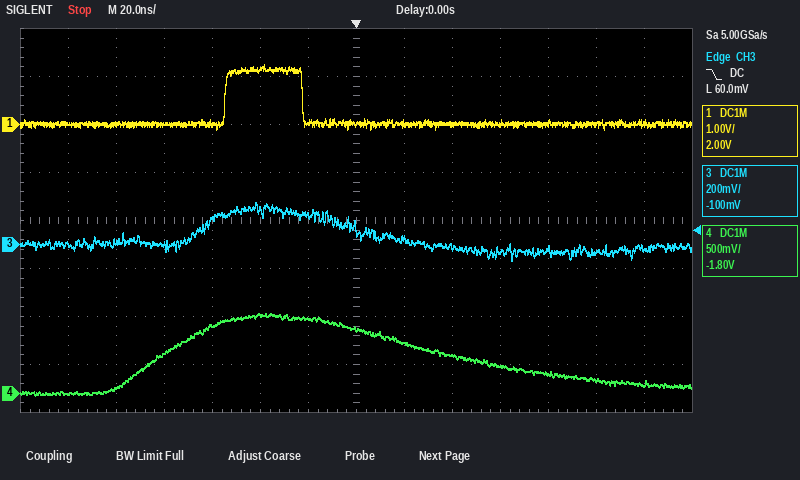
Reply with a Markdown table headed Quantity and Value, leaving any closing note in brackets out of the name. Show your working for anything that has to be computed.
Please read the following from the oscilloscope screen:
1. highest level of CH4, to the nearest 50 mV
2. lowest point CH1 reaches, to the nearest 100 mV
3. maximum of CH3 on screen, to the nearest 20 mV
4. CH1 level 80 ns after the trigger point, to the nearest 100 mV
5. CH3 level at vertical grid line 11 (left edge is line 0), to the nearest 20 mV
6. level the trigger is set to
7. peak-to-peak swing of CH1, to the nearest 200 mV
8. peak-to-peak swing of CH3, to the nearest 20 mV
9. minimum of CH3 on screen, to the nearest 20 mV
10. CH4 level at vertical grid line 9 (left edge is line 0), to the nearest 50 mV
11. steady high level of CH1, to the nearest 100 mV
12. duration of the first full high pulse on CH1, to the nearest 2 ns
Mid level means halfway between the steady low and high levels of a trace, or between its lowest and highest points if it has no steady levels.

| Quantity | Value |
|---|---|
| highest level of CH4, to the nearest 50 mV | 850 mV |
| lowest point CH1 reaches, to the nearest 100 mV | -100 mV |
| maximum of CH3 on screen, to the nearest 20 mV | 180 mV |
| CH1 level 80 ns after the trigger point, to the nearest 100 mV | 0.0 V |
| CH3 level at vertical grid line 11 (left edge is line 0), to the nearest 20 mV | -20 mV |
| level the trigger is set to | 60.0 mV |
| peak-to-peak swing of CH1, to the nearest 200 mV | 1.4 V |
| peak-to-peak swing of CH3, to the nearest 20 mV | 180 mV − (-60 mV) = 240 mV |
| minimum of CH3 on screen, to the nearest 20 mV | -60 mV |
| CH4 level at vertical grid line 9 (left edge is line 0), to the nearest 50 mV | 400 mV |
| steady high level of CH1, to the nearest 100 mV | 1.1 V |
| duration of the first full high pulse on CH1, to the nearest 2 ns | 32 ns |
